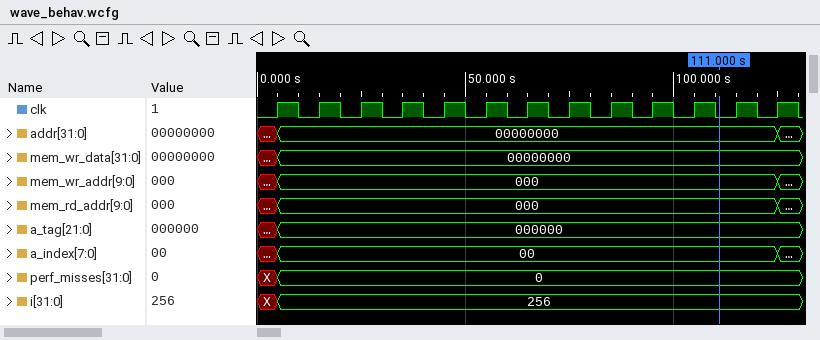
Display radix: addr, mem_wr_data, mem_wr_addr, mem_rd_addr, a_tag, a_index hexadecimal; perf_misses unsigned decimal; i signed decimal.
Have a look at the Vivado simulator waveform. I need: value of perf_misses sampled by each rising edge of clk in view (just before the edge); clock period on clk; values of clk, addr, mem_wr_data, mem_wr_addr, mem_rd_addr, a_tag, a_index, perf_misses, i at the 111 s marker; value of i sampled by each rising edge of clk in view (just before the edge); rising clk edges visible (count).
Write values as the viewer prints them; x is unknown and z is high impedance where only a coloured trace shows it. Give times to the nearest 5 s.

X, 0, 0, 0, 0, 0, 0, 0, 0, 0, 0, 0, 0
10 s
clk=0, addr=00000000, mem_wr_data=00000000, mem_wr_addr=000, mem_rd_addr=000, a_tag=000000, a_index=00, perf_misses=0, i=256
X, 256, 256, 256, 256, 256, 256, 256, 256, 256, 256, 256, 256
13
